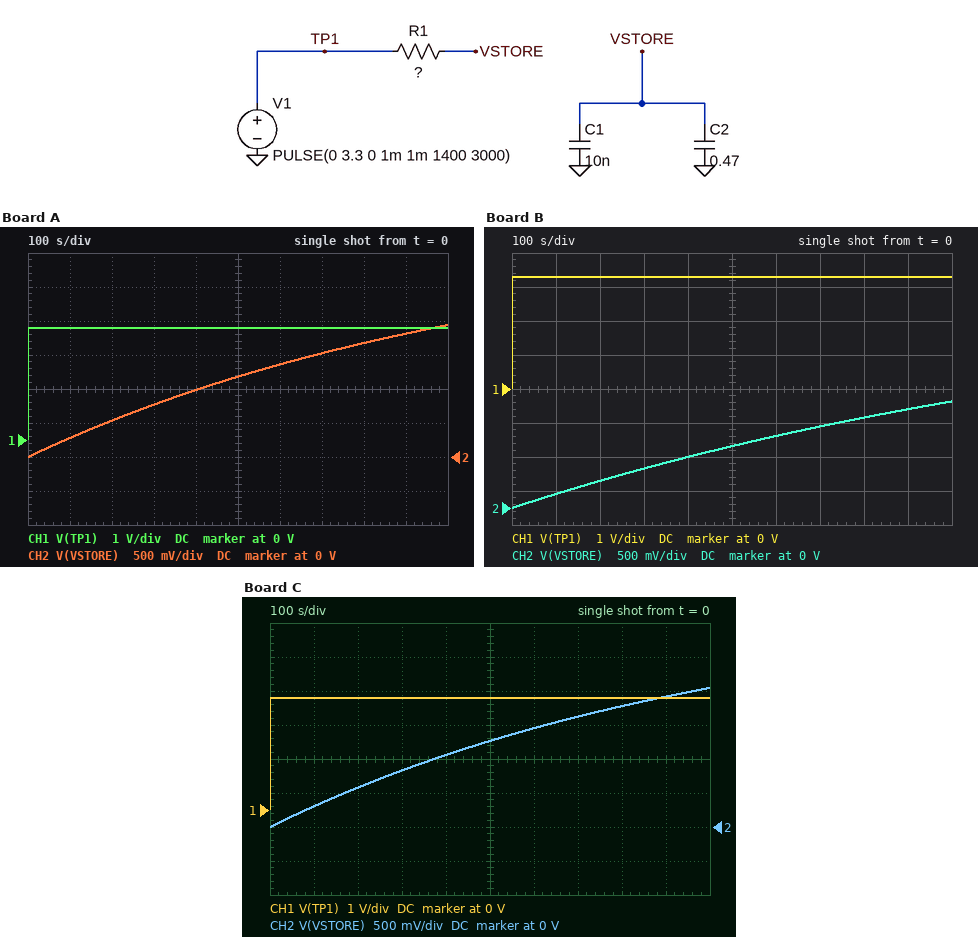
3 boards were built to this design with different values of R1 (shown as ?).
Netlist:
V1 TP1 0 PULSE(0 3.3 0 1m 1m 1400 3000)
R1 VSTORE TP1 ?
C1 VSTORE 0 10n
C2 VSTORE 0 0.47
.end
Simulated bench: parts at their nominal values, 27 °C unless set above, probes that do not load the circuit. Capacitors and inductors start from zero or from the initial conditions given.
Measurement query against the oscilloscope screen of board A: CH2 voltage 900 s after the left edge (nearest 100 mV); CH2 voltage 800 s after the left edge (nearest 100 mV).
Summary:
1.8 V
1.7 V
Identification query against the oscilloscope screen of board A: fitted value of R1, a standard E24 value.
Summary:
2.4 kΩ
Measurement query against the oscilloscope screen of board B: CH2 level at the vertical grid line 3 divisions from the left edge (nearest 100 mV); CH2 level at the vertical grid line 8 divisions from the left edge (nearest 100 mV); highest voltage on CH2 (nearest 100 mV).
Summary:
600 mV
1.3 V
1.6 V
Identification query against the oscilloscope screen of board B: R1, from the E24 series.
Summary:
3.3 kΩ
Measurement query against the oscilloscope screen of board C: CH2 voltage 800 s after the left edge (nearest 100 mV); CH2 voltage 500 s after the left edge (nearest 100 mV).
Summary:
1.8 V
1.3 V
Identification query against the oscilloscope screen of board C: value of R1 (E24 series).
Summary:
2.2 kΩ
